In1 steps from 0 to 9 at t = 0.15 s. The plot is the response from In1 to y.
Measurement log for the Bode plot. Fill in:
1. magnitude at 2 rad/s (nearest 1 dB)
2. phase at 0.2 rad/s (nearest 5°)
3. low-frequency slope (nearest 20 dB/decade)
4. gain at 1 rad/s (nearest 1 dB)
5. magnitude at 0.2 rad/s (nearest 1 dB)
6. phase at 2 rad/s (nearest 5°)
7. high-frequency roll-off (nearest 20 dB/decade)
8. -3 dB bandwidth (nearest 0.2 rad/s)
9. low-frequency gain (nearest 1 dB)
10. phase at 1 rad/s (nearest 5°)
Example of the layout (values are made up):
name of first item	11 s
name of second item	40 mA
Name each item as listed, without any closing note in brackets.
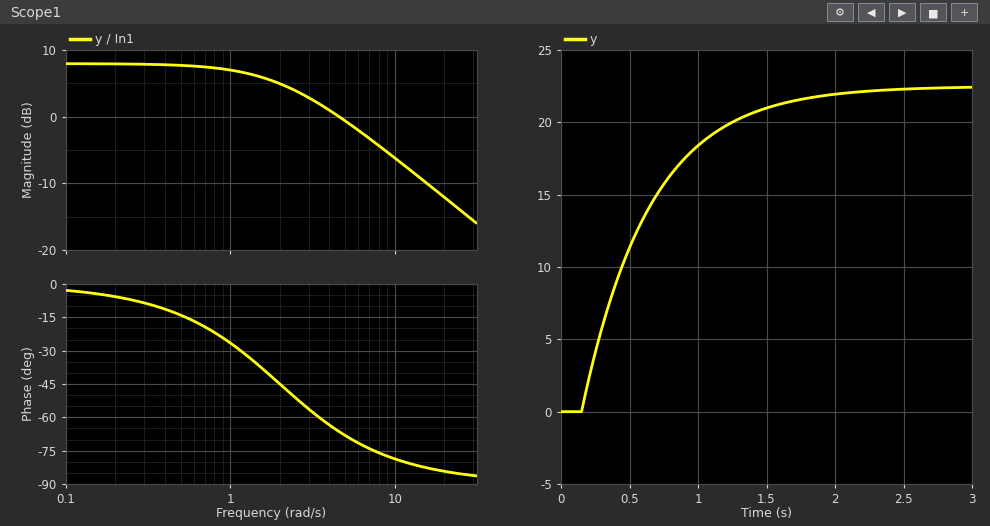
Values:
magnitude at 2 rad/s	5 dB
phase at 0.2 rad/s	-5°
low-frequency slope	0 dB/decade
gain at 1 rad/s	7 dB
magnitude at 0.2 rad/s	8 dB
phase at 2 rad/s	-45°
high-frequency roll-off	-20 dB/decade
-3 dB bandwidth	2.0 rad/s
low-frequency gain	8 dB
phase at 1 rad/s	-25°
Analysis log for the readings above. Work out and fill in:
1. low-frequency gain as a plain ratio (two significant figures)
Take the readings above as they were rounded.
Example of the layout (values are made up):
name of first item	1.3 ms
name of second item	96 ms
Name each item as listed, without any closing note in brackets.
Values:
low-frequency gain as a plain ratio	2.5
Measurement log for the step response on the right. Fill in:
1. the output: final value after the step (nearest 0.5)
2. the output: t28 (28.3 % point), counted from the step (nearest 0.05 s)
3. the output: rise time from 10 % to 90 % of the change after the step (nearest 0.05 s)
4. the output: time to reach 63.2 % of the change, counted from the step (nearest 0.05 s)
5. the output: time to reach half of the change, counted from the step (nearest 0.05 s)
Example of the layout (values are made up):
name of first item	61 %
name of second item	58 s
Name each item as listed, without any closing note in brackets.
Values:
the output: final value after the step	22.5
the output: t28 (28.3 % point), counted from the step	0.15 s
the output: rise time from 10 % to 90 % of the change after the step	1.10 s
the output: time to reach 63.2 % of the change, counted from the step	0.50 s
the output: time to reach half of the change, counted from the step	0.35 s
